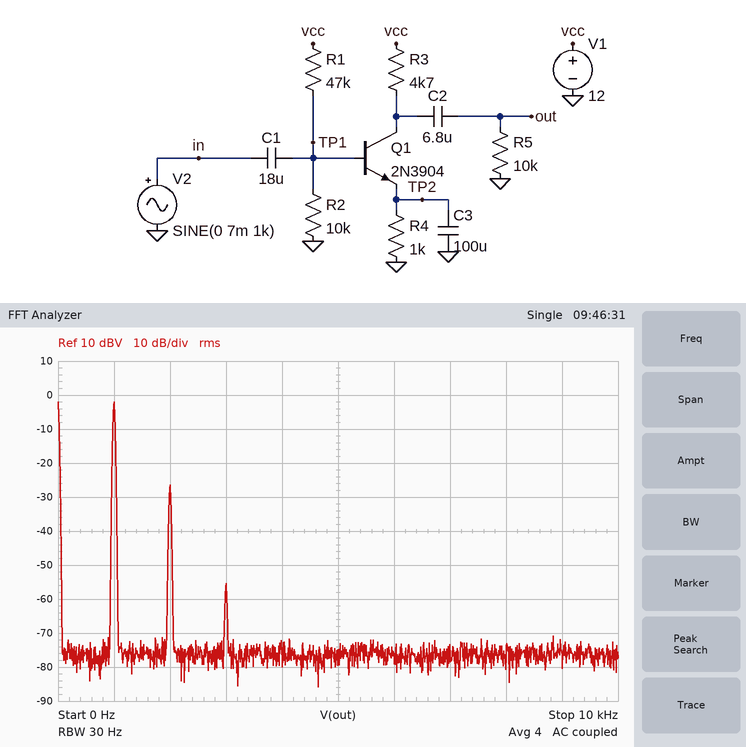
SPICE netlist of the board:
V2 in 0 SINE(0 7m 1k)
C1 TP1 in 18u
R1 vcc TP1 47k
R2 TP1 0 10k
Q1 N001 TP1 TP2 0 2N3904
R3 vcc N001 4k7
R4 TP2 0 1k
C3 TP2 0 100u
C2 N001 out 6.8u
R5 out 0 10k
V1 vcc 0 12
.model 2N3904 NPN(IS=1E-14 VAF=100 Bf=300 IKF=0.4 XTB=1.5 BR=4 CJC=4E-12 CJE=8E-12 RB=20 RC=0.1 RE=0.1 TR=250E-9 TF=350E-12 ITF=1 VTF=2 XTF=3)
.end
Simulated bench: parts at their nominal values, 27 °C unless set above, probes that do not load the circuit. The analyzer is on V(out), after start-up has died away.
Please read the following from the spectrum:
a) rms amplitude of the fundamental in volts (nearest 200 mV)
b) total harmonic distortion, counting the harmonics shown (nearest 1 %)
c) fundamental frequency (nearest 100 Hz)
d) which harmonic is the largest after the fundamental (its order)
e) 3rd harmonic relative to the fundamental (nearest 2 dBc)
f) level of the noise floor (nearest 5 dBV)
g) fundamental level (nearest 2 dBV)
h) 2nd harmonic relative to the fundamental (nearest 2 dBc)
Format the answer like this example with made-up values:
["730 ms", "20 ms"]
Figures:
["800 mV", "6 %", "1.0 kHz", "2", "-54 dBc", "-75 dBV", "-2 dBV", "-24 dBc"]
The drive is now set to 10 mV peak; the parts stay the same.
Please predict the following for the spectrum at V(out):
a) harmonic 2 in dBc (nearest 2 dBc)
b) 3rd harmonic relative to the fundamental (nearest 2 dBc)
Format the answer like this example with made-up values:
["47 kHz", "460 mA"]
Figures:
["-22 dBc", "-48 dBc"]
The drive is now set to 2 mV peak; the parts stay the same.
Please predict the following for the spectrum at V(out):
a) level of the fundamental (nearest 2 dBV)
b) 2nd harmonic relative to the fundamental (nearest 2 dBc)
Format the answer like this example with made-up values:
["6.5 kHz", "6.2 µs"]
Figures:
["-12 dBV", "-36 dBc"]
